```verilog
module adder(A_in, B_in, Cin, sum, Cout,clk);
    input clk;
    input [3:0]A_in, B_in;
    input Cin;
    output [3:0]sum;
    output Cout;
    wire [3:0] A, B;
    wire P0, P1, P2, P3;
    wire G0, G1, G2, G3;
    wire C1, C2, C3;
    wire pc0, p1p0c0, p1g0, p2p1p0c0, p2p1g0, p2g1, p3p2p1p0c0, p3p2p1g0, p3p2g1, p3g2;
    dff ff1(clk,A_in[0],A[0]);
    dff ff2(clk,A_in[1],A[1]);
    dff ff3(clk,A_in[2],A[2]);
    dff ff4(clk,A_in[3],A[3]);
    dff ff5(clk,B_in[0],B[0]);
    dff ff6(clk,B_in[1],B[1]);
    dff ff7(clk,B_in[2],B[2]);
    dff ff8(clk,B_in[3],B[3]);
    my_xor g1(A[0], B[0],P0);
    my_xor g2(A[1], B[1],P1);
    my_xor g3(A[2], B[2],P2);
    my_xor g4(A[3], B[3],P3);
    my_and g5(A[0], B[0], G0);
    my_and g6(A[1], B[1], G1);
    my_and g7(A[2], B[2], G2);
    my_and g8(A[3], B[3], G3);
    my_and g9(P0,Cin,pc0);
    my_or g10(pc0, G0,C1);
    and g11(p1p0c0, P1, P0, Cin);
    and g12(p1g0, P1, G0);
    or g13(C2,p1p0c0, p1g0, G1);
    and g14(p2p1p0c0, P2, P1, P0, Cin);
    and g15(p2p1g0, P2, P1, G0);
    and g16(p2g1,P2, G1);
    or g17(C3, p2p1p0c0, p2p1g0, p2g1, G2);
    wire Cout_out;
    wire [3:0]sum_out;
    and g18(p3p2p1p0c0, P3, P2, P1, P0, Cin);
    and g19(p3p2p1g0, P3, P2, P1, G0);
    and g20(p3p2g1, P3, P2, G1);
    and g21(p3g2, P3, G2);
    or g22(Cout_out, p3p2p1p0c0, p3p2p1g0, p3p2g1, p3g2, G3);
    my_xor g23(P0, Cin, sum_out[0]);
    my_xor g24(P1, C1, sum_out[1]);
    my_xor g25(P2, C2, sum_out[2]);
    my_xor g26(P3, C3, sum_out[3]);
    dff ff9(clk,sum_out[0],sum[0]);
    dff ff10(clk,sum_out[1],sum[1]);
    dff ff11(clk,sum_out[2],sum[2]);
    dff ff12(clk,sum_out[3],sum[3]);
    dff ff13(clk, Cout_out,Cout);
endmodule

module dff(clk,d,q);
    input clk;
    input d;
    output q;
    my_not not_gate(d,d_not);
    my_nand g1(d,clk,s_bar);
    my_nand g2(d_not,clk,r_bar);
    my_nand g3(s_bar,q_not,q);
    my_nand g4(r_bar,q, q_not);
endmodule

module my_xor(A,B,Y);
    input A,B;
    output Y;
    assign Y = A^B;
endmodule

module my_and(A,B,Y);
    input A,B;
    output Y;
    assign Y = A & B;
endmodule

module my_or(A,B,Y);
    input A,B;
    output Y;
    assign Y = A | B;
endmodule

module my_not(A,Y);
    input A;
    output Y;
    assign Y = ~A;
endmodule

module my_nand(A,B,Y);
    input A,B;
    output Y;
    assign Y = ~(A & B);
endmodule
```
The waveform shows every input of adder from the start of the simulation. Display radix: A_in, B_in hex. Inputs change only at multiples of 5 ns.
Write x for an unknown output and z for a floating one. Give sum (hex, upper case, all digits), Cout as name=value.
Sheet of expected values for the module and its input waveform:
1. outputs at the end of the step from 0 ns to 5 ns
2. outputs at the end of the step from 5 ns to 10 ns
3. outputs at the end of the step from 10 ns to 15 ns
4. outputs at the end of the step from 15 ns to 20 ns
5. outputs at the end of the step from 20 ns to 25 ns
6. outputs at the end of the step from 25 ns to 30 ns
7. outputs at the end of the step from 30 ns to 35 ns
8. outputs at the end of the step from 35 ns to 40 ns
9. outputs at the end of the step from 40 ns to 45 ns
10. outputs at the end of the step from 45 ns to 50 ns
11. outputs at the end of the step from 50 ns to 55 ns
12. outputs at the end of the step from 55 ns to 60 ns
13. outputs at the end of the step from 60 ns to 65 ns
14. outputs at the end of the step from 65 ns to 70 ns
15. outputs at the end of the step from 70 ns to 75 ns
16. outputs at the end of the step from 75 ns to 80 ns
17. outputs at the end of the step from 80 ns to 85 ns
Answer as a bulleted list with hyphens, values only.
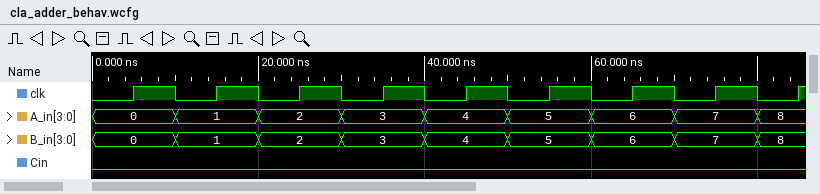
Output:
- sum=x, Cout=x
- sum=0, Cout=0
- sum=0, Cout=0
- sum=2, Cout=0
- sum=2, Cout=0
- sum=4, Cout=0
- sum=4, Cout=0
- sum=6, Cout=0
- sum=6, Cout=0
- sum=8, Cout=0
- sum=8, Cout=0
- sum=A, Cout=0
- sum=A, Cout=0
- sum=C, Cout=0
- sum=C, Cout=0
- sum=E, Cout=0
- sum=E, Cout=0
